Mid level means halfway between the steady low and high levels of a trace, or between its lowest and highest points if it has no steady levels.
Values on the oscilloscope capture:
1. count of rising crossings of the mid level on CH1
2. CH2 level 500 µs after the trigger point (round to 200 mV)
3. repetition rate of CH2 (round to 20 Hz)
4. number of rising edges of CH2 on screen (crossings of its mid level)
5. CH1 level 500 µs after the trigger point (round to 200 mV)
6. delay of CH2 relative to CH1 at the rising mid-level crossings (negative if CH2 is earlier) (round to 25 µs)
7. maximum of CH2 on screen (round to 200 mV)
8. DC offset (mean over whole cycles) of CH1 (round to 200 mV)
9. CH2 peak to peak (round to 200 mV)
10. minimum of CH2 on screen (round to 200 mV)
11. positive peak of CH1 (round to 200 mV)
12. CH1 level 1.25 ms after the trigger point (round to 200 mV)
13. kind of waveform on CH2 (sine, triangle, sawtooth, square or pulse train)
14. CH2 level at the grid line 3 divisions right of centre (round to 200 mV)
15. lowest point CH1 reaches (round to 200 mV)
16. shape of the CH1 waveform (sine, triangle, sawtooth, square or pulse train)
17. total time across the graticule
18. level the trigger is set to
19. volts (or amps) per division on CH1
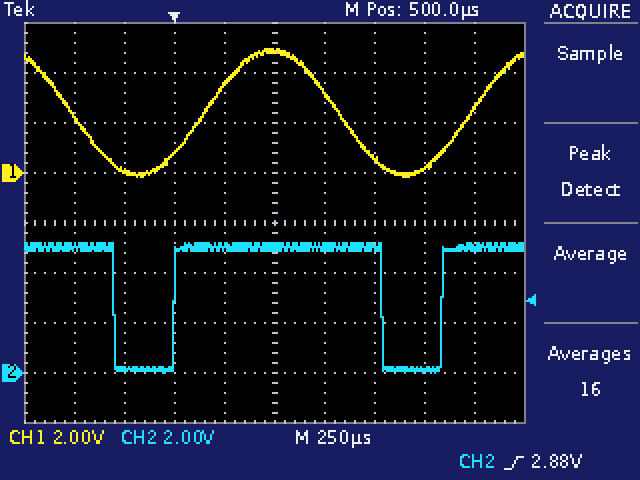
2
5.0 V
740 Hz
2
4.8 V
-150 µs
5.2 V
2.4 V
5.2 V
0.0 V
5.0 V
200 mV
pulse train
200 mV
-200 mV
sine
2.5 ms
2.88 V
2 V
